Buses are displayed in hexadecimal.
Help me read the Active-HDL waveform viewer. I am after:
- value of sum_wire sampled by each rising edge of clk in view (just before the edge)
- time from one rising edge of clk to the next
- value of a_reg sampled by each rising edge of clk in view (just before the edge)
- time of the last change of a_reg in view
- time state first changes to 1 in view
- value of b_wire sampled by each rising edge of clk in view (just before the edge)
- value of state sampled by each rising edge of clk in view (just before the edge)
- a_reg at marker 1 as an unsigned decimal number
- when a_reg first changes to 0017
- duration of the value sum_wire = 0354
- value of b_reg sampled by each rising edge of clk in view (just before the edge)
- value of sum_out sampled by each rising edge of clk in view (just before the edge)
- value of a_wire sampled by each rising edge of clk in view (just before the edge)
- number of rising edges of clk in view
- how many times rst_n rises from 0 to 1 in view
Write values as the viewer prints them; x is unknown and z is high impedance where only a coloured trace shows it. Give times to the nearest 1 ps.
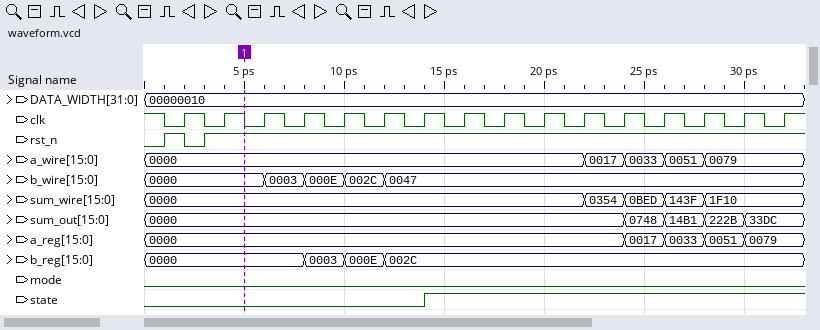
0000, 0000, 0000, 0000, 0000, 0000, 0000, 0000, 0000, 0000, 0000, 0354, 0BED, 143F, 1F10, 1F10
2 ps
0000, 0000, 0000, 0000, 0000, 0000, 0000, 0000, 0000, 0000, 0000, 0000, 0017, 0033, 0051, 0079
30 ps
14 ps
0000, 0000, 0000, 0003, 000E, 002C, 0047, 0047, 0047, 0047, 0047, 0047, 0047, 0047, 0047, 0047
0 0 0 0 0 0 0 1 1 1 1 1 1 1 1 1
0
24 ps
2 ps
0000, 0000, 0000, 0000, 0003, 000E, 002C, 002C, 002C, 002C, 002C, 002C, 002C, 002C, 002C, 002C
0000, 0000, 0000, 0000, 0000, 0000, 0000, 0000, 0000, 0000, 0000, 0000, 0748, 14B1, 222B, 33DC
0000, 0000, 0000, 0000, 0000, 0000, 0000, 0000, 0000, 0000, 0000, 0017, 0033, 0051, 0079, 0079
16
2
